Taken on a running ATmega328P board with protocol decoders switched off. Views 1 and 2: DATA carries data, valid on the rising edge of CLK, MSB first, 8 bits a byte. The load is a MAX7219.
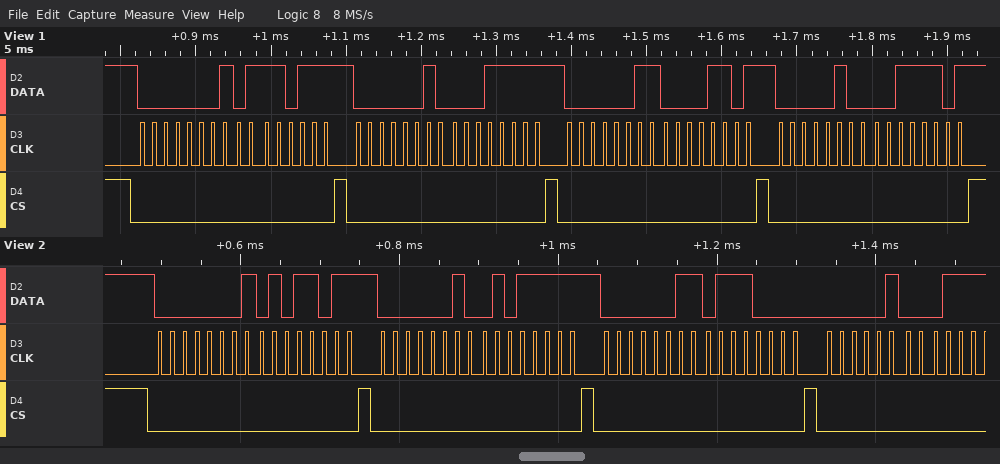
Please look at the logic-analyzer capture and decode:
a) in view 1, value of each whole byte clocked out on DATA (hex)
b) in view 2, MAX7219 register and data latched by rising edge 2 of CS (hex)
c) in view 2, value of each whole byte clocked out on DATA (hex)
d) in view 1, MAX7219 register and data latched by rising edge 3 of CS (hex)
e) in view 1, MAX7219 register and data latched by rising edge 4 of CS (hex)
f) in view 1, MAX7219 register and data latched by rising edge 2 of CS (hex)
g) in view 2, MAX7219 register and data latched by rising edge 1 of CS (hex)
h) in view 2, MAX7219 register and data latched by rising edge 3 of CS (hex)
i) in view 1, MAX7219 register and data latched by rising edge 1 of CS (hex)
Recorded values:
01 77 02 1F 03 0D 04 3D
register 0x2, data 0x5F
01 5B 02 5F 03 70 04
register 0x3, data 0x0D
register 0x4, data 0x3D
register 0x2, data 0x1F
register 0x1, data 0x5B
register 0x3, data 0x70
register 0x1, data 0x77
